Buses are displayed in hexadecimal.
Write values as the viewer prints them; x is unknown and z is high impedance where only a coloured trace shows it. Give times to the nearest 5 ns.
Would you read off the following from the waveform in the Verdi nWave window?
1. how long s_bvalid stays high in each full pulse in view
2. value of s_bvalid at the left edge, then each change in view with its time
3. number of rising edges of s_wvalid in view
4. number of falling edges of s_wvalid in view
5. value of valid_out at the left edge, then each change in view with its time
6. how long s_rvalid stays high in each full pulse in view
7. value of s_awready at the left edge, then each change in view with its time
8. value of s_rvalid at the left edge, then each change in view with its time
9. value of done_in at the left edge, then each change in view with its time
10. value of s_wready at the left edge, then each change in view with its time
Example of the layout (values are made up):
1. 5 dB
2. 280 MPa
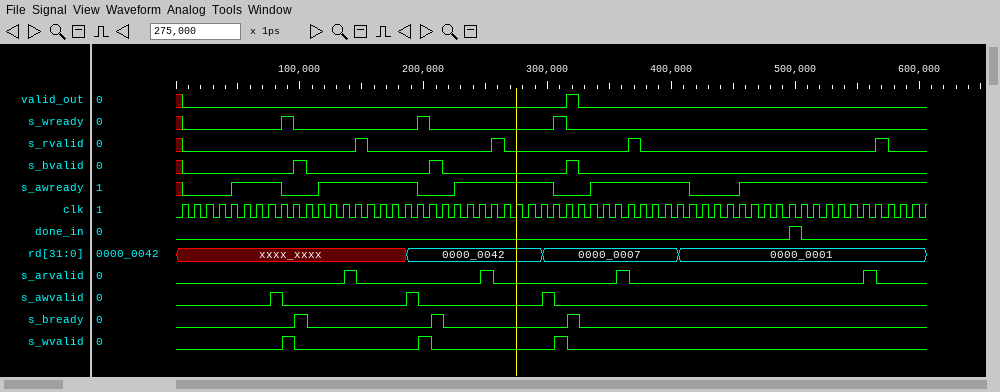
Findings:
1. 10 ns, 10 ns, 10 ns
2. x, 0 at 5 ns, 1 at 95 ns, 0 at 105 ns, 1 at 205 ns, 0 at 215 ns, 1 at 315 ns, 0 at 325 ns
3. 3
4. 3
5. x, 0 at 5 ns, 1 at 315 ns, 0 at 325 ns
6. 10 ns, 10 ns, 10 ns, 10 ns
7. x, 0 at 5 ns, 1 at 45 ns, 0 at 85 ns, 1 at 115 ns, 0 at 195 ns, 1 at 225 ns, 0 at 305 ns, 1 at 335 ns, 0 at 415 ns, 1 at 455 ns
8. x, 0 at 5 ns, 1 at 145 ns, 0 at 155 ns, 1 at 255 ns, 0 at 265 ns, 1 at 365 ns, 0 at 375 ns, 1 at 565 ns, 0 at 575 ns
9. 0, 1 at 495 ns, 0 at 505 ns
10. x, 0 at 5 ns, 1 at 85 ns, 0 at 95 ns, 1 at 195 ns, 0 at 205 ns, 1 at 305 ns, 0 at 315 ns
